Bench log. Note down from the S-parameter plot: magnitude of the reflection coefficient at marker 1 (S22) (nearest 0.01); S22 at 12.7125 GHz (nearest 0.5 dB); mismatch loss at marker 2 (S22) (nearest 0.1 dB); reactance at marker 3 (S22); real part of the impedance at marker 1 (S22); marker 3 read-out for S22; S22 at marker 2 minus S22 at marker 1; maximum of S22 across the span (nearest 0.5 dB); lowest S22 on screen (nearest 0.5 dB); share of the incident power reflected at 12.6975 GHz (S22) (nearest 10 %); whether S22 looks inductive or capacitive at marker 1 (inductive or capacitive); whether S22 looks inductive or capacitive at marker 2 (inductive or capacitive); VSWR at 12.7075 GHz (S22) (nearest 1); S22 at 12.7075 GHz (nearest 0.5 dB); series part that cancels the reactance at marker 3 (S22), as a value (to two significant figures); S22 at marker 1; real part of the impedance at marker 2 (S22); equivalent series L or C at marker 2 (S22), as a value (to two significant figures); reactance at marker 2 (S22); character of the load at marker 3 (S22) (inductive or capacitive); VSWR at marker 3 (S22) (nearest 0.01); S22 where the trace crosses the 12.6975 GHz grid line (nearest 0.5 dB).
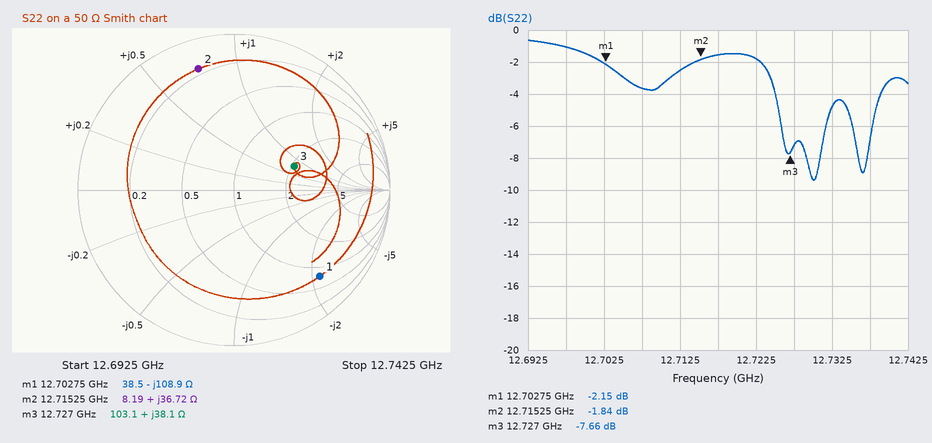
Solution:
0.78
-2.5 dB
4.6 dB
+38.1 Ω
38.5 Ω
-7.66 dB
0.31 dB
-0.5 dB
-9.5 dB
80 %
capacitive
inductive
5
-3.5 dB
330 fF
-2.15 dB
8.19 Ω
460 pH
+36.72 Ω
inductive
2.41
-1.0 dB
